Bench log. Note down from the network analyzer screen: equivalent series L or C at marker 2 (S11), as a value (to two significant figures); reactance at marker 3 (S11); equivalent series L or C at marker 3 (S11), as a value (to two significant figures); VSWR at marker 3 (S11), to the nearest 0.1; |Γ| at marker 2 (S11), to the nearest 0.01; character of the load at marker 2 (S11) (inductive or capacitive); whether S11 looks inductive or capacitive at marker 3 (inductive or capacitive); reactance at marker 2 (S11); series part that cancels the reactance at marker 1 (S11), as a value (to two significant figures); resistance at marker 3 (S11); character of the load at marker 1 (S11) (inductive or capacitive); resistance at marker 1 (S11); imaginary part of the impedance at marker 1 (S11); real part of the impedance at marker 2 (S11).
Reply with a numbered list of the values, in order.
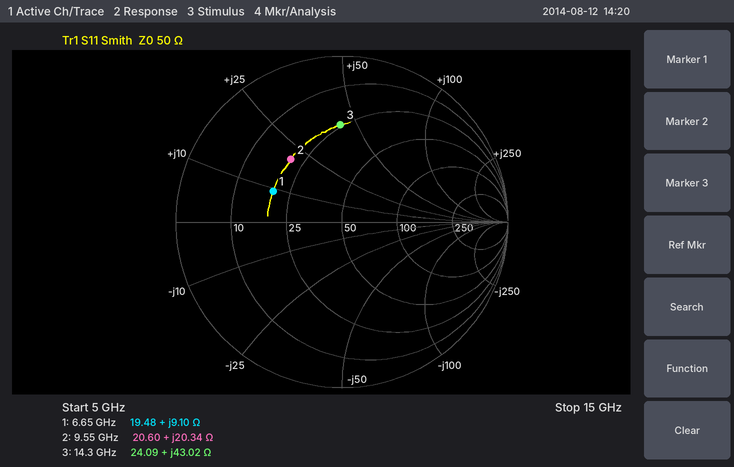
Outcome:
1. 340 pH
2. +43.02 Ω
3. 480 pH
4. 3.8
5. 0.49
6. inductive
7. inductive
8. +20.34 Ω
9. 2.6 pF
10. 24.09 Ω
11. inductive
12. 19.48 Ω
13. +9.10 Ω
14. 20.60 Ω
